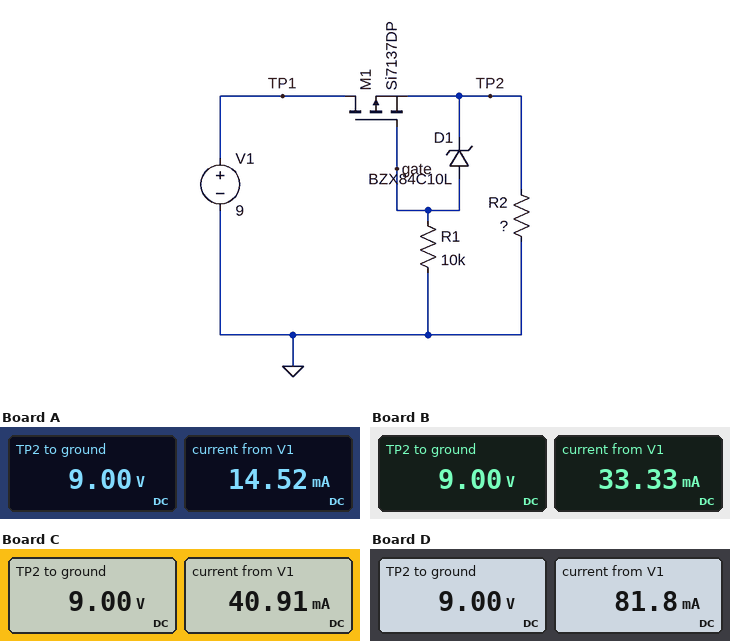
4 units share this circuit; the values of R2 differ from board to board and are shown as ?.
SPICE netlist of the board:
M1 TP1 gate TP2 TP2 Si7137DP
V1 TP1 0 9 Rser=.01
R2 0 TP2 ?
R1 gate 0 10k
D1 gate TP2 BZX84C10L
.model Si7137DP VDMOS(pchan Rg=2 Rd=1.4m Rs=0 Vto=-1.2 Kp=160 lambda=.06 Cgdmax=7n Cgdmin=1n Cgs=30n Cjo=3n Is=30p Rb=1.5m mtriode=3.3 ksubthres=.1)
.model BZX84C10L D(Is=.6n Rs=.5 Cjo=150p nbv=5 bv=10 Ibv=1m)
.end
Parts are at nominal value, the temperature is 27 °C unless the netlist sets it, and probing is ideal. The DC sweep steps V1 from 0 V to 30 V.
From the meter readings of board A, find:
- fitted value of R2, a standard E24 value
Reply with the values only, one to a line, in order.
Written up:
620 Ω
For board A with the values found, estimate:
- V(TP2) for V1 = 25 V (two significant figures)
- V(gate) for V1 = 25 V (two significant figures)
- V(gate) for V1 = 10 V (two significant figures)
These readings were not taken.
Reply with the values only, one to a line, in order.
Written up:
25 V
15 V
410 mV
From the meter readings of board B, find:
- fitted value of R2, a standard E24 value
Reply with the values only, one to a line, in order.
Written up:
270 Ω
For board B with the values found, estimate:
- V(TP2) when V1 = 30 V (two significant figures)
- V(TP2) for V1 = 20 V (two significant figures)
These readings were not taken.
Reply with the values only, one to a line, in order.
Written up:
30 V
20 V
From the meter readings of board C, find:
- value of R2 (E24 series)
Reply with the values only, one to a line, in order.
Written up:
220 Ω
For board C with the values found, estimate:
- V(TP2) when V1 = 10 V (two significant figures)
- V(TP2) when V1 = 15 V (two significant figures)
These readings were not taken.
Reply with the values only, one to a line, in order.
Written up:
10 V
15 V
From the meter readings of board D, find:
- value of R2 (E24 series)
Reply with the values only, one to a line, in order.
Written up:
110 Ω
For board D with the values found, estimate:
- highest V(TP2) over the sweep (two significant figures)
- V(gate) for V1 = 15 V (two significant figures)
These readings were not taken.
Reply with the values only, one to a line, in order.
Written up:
30 V
5.1 V
